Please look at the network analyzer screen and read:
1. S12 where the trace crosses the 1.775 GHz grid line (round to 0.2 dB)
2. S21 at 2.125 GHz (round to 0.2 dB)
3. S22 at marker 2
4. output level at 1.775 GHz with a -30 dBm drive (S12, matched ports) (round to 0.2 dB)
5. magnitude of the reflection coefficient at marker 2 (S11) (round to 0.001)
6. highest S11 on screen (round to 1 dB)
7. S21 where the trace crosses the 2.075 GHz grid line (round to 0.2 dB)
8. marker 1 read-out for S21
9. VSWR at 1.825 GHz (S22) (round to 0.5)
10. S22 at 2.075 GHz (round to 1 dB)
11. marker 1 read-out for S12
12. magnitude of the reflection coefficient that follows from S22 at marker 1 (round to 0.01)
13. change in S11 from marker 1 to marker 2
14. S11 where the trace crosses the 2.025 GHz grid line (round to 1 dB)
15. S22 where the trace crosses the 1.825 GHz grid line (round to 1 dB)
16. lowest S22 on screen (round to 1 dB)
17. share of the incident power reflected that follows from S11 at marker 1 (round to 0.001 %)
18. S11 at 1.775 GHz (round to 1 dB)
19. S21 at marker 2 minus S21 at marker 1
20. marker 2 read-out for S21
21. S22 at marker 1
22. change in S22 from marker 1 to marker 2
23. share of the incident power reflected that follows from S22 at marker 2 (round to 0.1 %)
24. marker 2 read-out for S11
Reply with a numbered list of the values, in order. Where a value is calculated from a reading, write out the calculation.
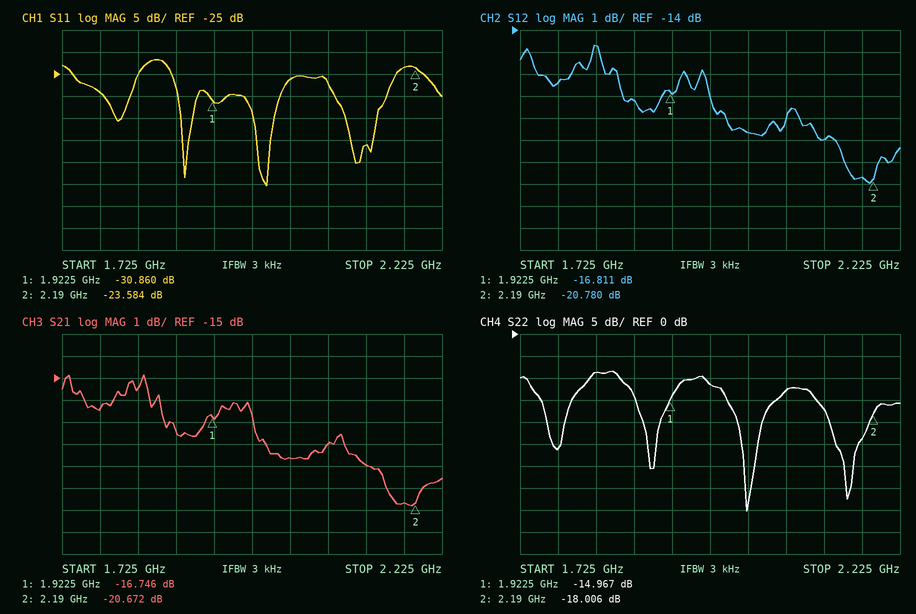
1. -16.4 dB
2. -19.0 dB
3. -18.006 dB
4. -30 dBm + (-16.4 dB) = -46.4 dBm
5. 10^(-23.584/20) ≈ 0.066
6. -22 dB
7. -18.0 dB
8. -16.746 dB
9. |Γ| = 10^(-9/20) = 0.3548; VSWR = (1 + 0.3548)/(1 − 0.3548) ≈ 2.10, so 2.0 to the nearest 0.5
10. -13 dB
11. -16.811 dB
12. 10^(-14.967/20) ≈ 0.18
13. -23.584 − (-30.86) = 7.276 dB
14. -26 dB
15. -9 dB
16. -40 dB
17. 10^(-30.86/10) ≈ 0.082 %
18. -29 dB
19. -20.672 − (-16.746) = -3.926 dB
20. -20.672 dB
21. -14.967 dB
22. -18.006 − (-14.967) = -3.039 dB
23. 10^(-18.006/10) ≈ 1.6 %
24. -23.584 dB
